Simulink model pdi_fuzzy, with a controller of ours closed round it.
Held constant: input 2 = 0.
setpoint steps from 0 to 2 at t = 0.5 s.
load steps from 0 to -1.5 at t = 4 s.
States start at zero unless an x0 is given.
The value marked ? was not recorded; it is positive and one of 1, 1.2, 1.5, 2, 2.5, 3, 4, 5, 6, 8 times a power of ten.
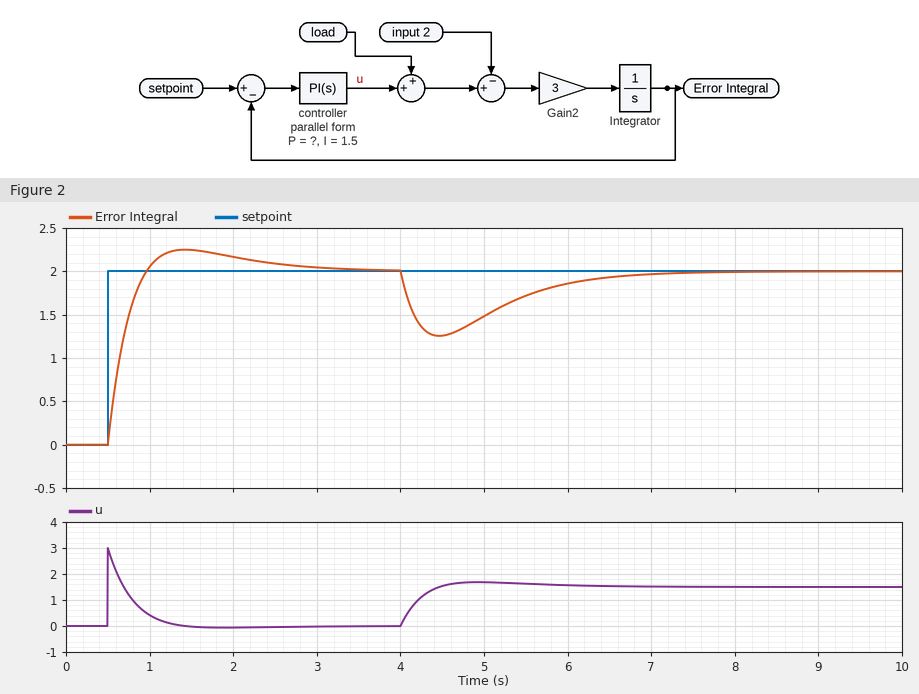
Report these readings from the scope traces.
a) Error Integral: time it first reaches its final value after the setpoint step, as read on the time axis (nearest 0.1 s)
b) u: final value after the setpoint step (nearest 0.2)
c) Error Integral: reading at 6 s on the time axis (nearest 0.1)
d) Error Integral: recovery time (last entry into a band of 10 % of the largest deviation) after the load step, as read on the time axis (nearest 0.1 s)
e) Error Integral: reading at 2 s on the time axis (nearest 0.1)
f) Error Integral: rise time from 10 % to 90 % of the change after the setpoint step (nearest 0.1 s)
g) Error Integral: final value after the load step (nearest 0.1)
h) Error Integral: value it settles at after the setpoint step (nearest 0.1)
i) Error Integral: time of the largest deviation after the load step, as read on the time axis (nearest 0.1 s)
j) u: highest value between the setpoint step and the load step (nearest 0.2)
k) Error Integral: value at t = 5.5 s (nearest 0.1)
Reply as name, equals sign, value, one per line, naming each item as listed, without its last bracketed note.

Error Integral: time it first reaches its final value after the setpoint step, as read on the time axis = 1.0 s
u: final value after the setpoint step = 0.0
Error Integral: reading at 6 s on the time axis = 1.9
Error Integral: recovery time (last entry into a band of 10 % of the largest deviation) after the load step, as read on the time axis = 6.4 s
Error Integral: reading at 2 s on the time axis = 2.2
Error Integral: rise time from 10 % to 90 % of the change after the setpoint step = 0.3 s
Error Integral: final value after the load step = 2.0
Error Integral: value it settles at after the setpoint step = 2.0
Error Integral: time of the largest deviation after the load step, as read on the time axis = 4.5 s
u: highest value between the setpoint step and the load step = 3.0
Error Integral: value at t = 5.5 s = 1.7
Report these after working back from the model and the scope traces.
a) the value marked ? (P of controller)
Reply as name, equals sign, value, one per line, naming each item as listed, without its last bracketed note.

the value marked ? = 1.5
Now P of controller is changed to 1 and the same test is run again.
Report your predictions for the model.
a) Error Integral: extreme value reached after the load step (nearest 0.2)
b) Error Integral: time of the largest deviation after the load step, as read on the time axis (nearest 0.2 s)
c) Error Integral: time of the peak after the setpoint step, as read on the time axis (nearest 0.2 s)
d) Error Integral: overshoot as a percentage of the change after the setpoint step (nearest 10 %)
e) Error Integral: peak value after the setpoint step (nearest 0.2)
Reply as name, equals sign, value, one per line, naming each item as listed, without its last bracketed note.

Error Integral: extreme value reached after the load step = 1.0
Error Integral: time of the largest deviation after the load step, as read on the time axis = 4.6 s
Error Integral: time of the peak after the setpoint step, as read on the time axis = 1.6 s
Error Integral: overshoot as a percentage of the change after the setpoint step = 20 %
Error Integral: peak value after the setpoint step = 2.4
